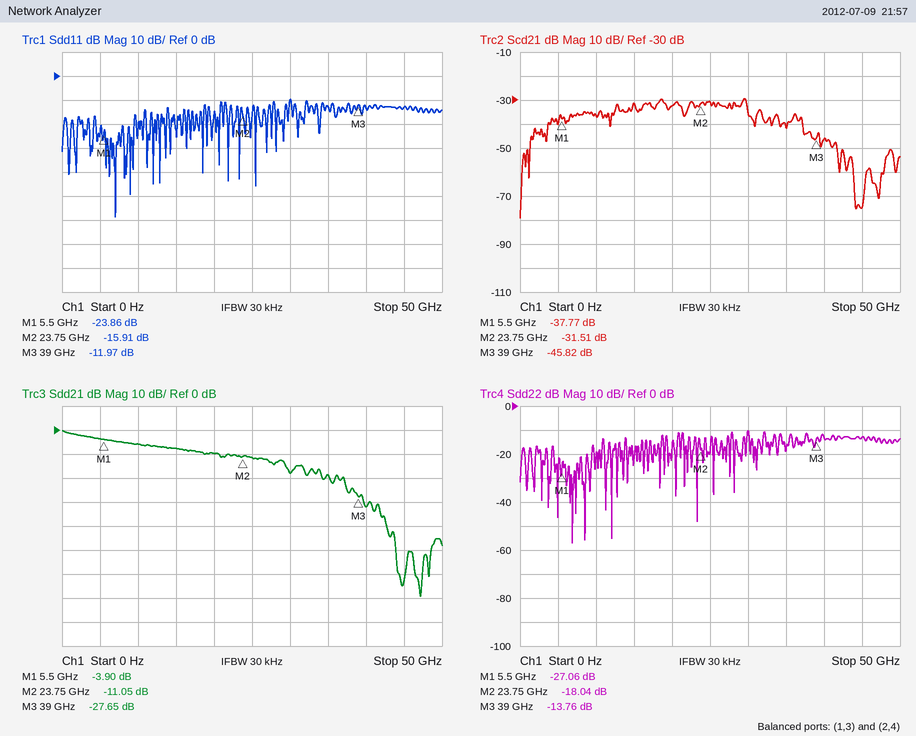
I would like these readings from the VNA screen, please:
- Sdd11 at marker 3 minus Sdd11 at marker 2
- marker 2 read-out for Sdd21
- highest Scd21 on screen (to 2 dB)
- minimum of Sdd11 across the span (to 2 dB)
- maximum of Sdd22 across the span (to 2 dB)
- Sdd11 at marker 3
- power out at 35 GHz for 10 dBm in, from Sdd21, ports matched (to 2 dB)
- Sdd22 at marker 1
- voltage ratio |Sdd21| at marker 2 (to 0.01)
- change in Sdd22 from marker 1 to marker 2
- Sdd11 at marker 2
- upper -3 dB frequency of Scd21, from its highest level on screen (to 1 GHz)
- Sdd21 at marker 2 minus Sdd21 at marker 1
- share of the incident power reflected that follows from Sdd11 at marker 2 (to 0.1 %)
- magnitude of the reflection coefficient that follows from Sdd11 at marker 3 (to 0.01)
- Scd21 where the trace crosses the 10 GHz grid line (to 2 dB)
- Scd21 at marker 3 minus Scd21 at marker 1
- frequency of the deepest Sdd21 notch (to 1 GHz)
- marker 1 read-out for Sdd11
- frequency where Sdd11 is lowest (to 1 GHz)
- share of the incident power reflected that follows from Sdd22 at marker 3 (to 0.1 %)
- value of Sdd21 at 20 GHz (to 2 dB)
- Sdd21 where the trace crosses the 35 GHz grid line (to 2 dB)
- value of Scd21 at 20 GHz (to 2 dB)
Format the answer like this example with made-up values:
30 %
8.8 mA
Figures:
3.94 dB
-11.05 dB
-30 dB
-58 dB
-10 dB
-11.97 dB
-8 dBm
-27.06 dB
0.28
9.02 dB
-15.91 dB
30 GHz
-7.15 dB
2.6 %
0.25
-36 dB
-8.05 dB
47 GHz
-23.86 dB
7 GHz
4.2 %
-10 dB
-18 dB
-32 dB
